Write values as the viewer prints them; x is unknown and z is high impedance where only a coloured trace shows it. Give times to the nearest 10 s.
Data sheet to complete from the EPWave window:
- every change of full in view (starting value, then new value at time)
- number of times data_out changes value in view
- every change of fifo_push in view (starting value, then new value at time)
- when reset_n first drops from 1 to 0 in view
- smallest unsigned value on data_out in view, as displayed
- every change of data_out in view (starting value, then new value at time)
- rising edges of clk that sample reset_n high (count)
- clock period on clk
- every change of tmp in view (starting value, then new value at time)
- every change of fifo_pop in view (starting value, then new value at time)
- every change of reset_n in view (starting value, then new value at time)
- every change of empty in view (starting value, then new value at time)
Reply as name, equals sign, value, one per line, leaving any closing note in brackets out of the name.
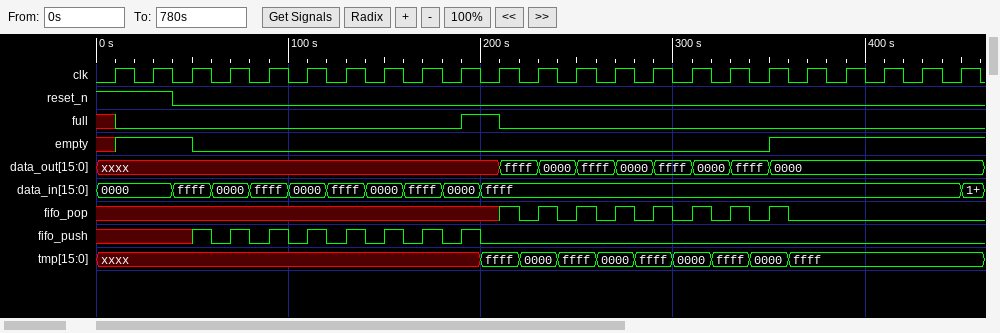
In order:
every change of full in view = x, 0 at 10 s, 1 at 190 s, 0 at 210 s
number of times data_out changes value in view = 8
every change of fifo_push in view = x, 1 at 50 s, 0 at 60 s, 1 at 70 s, 0 at 80 s, 1 at 90 s, 0 at 100 s, 1 at 110 s, 0 at 120 s, 1 at 130 s, 0 at 140 s, 1 at 150 s, 0 at 160 s, 1 at 170 s, 0 at 180 s, 1 at 190 s, 0 at 200 s
when reset_n first drops from 1 to 0 in view = 40 s
smallest unsigned value on data_out in view, as displayed = 0000
every change of data_out in view = xxxx, ffff at 210 s, 0000 at 230 s, ffff at 250 s, 0000 at 270 s, ffff at 290 s, 0000 at 310 s, ffff at 330 s, 0000 at 350 s
rising edges of clk that sample reset_n high = 2
clock period on clk = 20 s
every change of tmp in view = xxxx, ffff at 200 s, 0000 at 220 s, ffff at 240 s, 0000 at 260 s, ffff at 280 s, 0000 at 300 s, ffff at 320 s, 0000 at 340 s, ffff at 360 s
every change of fifo_pop in view = x, 1 at 210 s, 0 at 220 s, 1 at 230 s, 0 at 240 s, 1 at 250 s, 0 at 260 s, 1 at 270 s, 0 at 280 s, 1 at 290 s, 0 at 300 s, 1 at 310 s, 0 at 320 s, 1 at 330 s, 0 at 340 s, 1 at 350 s, 0 at 360 s
every change of reset_n in view = 1, 0 at 40 s
every change of empty in view = x, 1 at 10 s, 0 at 50 s, 1 at 350 s
